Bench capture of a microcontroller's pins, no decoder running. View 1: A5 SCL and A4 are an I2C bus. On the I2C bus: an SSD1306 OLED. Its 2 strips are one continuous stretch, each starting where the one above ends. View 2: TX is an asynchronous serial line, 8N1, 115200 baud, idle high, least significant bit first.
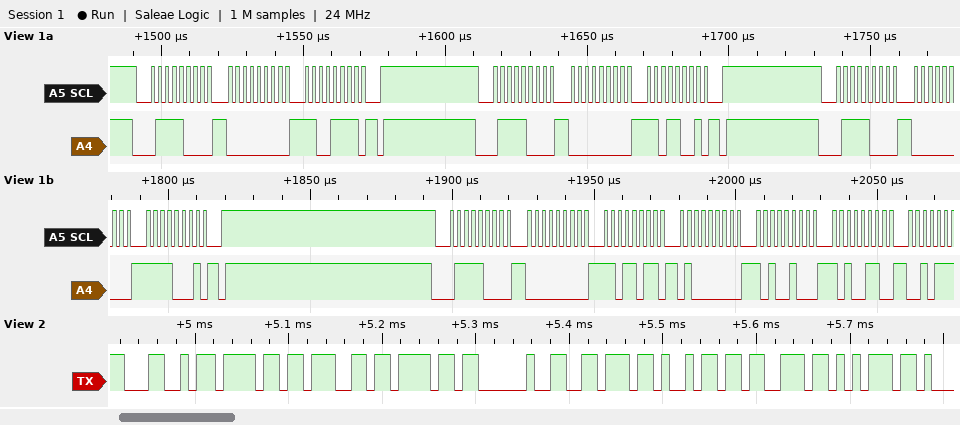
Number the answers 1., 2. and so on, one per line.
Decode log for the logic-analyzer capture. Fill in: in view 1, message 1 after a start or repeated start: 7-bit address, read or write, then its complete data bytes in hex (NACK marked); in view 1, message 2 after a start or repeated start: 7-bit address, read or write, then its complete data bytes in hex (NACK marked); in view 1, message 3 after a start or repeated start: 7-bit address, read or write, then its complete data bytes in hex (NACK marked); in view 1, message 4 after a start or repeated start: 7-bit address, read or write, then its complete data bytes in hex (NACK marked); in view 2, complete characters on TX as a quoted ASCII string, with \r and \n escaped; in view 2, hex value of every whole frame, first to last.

1. 0x3C write: 00 CF
2. 0x3C write: 00 D9
3. 0x3C write: 00 F1
4. 0x3C write: 00 DB 40 A4 A6
5. "Logo visu"
6. 0x4C 0x6F 0x67 0x6F 0x20 0x76 0x69 0x73 0x75
